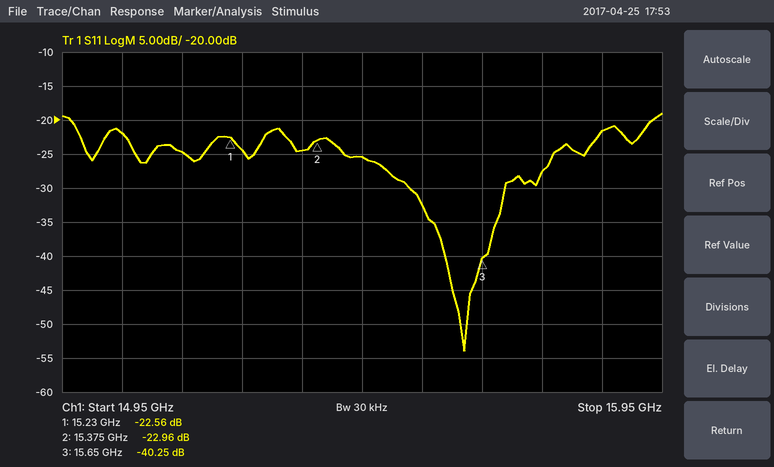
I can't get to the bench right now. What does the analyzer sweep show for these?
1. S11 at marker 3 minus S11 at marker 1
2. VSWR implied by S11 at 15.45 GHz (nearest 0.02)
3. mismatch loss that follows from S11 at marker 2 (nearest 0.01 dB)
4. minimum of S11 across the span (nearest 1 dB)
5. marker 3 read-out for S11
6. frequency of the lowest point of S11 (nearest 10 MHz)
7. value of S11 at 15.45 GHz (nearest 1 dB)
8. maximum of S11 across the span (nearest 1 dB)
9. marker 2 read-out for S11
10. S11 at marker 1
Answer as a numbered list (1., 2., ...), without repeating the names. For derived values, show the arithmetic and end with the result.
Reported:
1. -40.25 − (-22.56) = -17.69 dB
2. |Γ| = 10^(-25/20) = 0.0562; VSWR = (1 + 0.0562)/(1 − 0.0562) ≈ 1.12
3. −10 log10(1 − 10^(-22.96/10)) ≈ 0.02 dB
4. -54 dB
5. -40.25 dB
6. 15.62 GHz
7. -25 dB
8. -19 dB
9. -22.96 dB
10. -22.56 dB
